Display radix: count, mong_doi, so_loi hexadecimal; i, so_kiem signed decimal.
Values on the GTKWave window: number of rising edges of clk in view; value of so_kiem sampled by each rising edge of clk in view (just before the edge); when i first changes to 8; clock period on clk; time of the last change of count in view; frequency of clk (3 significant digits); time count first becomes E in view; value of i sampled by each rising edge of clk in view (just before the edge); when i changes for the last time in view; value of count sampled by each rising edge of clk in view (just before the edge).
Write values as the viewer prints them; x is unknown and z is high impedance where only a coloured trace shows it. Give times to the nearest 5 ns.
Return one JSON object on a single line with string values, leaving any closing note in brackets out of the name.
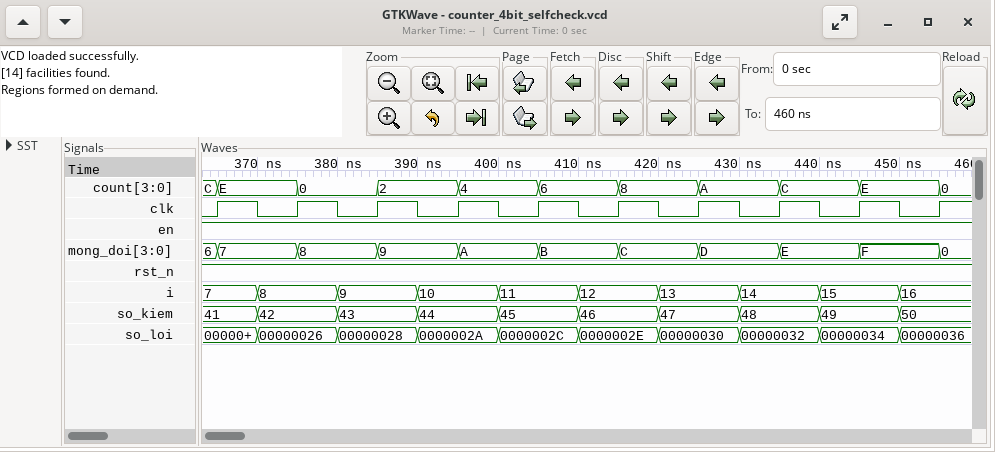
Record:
{"number of rising edges of clk in view": "10", "value of so_kiem sampled by each rising edge of clk in view": "41, 42, 43, 44, 45, 46, 47, 48, 49, 50", "when i first changes to 8": "370 ns", "clock period on clk": "10 ns", "time of the last change of count in view": "455 ns", "frequency of clk": "100 MHz", "time count first becomes E in view": "365 ns", "value of i sampled by each rising edge of clk in view": "7, 8, 9, 10, 11, 12, 13, 14, 15, 16", "when i changes for the last time in view": "450 ns", "value of count sampled by each rising edge of clk in view": "C, E, 0, 2, 4, 6, 8, A, C, E"}
